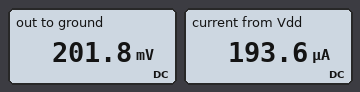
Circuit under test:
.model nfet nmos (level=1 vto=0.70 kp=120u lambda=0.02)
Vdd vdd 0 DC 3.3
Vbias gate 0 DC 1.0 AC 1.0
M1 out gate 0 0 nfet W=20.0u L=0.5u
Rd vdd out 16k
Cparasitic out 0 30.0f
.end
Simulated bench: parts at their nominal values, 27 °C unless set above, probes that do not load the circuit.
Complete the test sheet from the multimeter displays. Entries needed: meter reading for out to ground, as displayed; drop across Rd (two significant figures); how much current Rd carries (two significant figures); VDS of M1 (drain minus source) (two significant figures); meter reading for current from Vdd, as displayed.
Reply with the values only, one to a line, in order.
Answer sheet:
201.8 mV
3.1 V
190 µA
200 mV
193.6 µA
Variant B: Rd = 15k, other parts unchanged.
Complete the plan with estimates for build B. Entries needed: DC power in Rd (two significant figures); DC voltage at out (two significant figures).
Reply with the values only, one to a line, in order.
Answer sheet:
630 µW
230 mV
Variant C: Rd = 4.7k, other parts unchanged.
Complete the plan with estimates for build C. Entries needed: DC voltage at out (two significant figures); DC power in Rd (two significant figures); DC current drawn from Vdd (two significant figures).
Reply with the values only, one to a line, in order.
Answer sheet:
2.2 V
240 µW
230 µA
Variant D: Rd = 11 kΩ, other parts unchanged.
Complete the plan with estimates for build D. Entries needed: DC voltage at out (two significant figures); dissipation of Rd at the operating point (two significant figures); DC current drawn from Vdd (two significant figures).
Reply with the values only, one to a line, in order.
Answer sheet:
880 mV
530 µW
220 µA
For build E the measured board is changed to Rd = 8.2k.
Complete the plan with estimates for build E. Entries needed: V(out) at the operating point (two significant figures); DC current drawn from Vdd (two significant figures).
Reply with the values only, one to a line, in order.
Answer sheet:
1.5 V
220 µA
